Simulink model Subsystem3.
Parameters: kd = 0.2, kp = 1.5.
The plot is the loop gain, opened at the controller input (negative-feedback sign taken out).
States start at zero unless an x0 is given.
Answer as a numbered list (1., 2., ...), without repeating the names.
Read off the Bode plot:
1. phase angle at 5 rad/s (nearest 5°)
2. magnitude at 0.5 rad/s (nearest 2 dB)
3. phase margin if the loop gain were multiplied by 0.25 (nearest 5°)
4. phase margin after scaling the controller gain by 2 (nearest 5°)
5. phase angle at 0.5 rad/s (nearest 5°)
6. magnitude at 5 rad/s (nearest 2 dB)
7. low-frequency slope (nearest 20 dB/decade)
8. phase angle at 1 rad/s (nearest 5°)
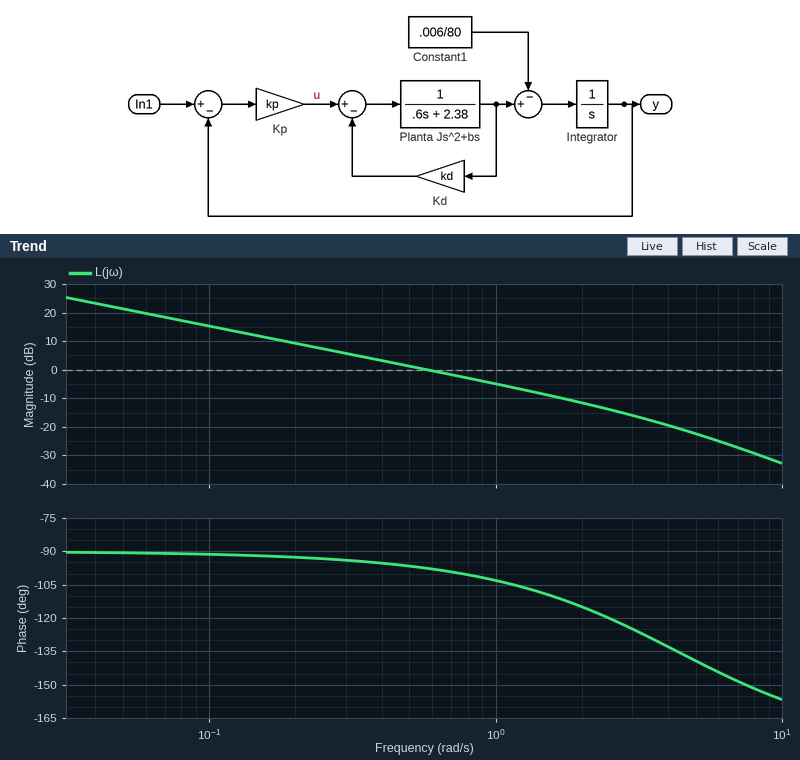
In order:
1. -140°
2. 2 dB
3. 90°
4. 75°
5. -95°
6. -22 dB
7. -20 dB/decade
8. -105°
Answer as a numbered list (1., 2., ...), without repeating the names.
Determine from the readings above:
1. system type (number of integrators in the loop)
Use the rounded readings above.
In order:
1. 1
